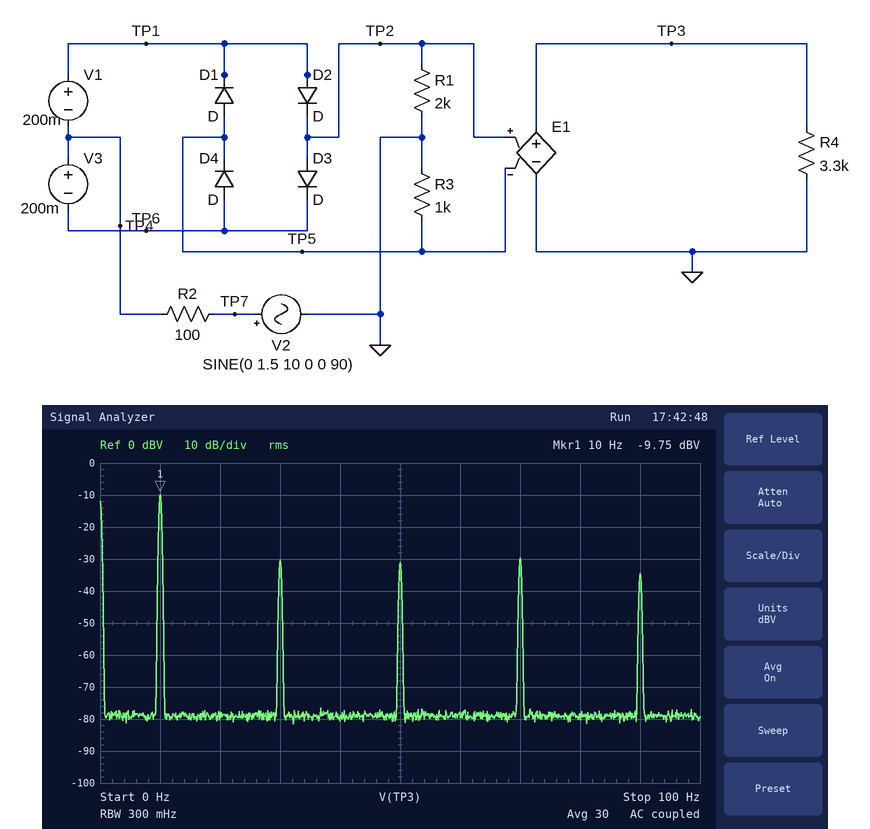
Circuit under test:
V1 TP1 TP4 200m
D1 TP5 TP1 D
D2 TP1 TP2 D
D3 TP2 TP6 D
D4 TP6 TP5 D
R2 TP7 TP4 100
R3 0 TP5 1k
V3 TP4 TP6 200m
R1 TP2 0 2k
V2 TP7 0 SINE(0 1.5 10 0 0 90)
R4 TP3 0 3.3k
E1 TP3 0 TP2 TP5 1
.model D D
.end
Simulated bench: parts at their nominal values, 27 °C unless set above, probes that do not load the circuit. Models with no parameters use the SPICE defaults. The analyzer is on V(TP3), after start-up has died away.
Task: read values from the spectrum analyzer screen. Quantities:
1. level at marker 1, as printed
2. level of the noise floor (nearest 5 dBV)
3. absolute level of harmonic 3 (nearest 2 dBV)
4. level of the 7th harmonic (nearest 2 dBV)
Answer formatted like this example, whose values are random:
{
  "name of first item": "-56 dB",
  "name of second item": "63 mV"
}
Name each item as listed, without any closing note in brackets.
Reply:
{
  "level at marker 1, as printed": "-9.75 dBV",
  "level of the noise floor": "-80 dBV",
  "absolute level of harmonic 3": "-30 dBV",
  "level of the 7th harmonic": "-30 dBV"
}
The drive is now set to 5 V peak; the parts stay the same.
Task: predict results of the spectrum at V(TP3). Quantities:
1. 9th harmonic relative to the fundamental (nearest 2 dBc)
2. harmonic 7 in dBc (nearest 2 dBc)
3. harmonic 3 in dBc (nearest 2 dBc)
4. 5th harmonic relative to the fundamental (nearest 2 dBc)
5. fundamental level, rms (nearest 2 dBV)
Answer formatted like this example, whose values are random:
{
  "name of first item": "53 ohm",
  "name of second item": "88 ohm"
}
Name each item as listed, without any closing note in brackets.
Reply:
{
  "9th harmonic relative to the fundamental": "-28 dBc",
  "harmonic 7 in dBc": "-22 dBc",
  "harmonic 3 in dBc": "-10 dBc",
  "5th harmonic relative to the fundamental": "-16 dBc",
  "fundamental level, rms": "-8 dBV"
}
